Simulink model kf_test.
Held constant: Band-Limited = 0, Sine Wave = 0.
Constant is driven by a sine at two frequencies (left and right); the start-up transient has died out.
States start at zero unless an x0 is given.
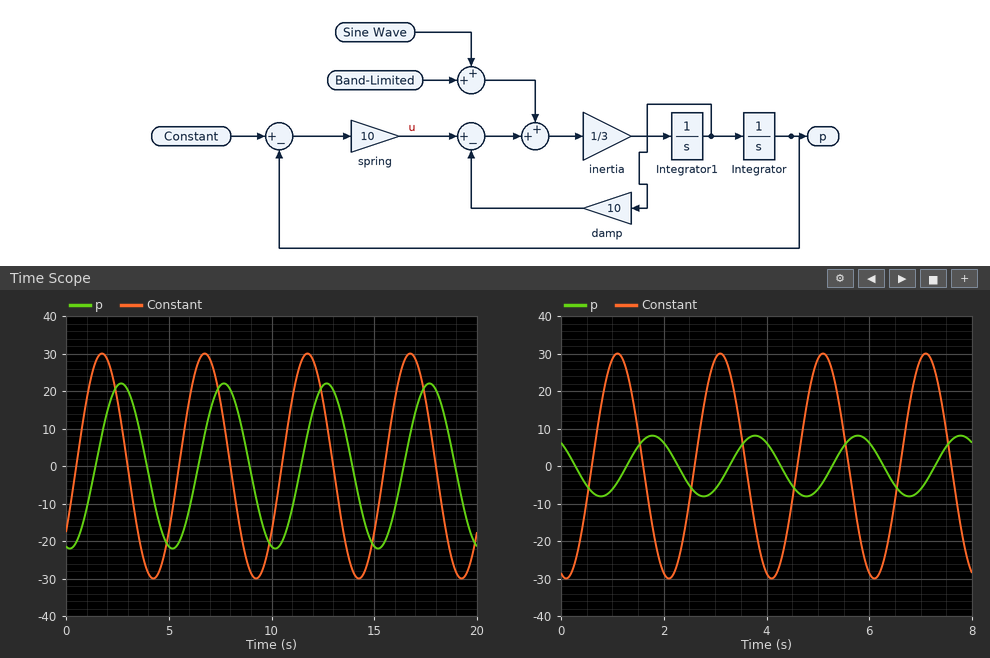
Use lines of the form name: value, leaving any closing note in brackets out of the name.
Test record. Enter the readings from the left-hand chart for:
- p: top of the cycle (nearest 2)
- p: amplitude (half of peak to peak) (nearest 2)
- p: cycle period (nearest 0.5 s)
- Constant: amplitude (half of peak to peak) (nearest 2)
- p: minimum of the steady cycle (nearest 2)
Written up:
p: top of the cycle: 22
p: amplitude (half of peak to peak): 22
p: cycle period: 5.0 s
Constant: amplitude (half of peak to peak): 30
p: minimum of the steady cycle: -22
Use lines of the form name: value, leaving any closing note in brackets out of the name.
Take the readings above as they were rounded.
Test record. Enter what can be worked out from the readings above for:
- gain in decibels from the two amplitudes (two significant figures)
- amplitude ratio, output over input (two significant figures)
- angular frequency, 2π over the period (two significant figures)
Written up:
gain in decibels from the two amplitudes: -2.7 dB
amplitude ratio, output over input: 0.73
angular frequency, 2π over the period: 1.3 rad/s
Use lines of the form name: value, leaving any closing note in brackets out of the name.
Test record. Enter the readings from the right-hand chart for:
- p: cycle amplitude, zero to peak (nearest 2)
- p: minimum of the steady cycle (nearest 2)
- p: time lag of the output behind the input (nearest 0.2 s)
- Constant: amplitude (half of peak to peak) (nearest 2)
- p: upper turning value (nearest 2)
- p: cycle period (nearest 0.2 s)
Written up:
p: cycle amplitude, zero to peak: 8
p: minimum of the steady cycle: -8
p: time lag of the output behind the input: 0.6 s
Constant: amplitude (half of peak to peak): 30
p: upper turning value: 8
p: cycle period: 2.0 s
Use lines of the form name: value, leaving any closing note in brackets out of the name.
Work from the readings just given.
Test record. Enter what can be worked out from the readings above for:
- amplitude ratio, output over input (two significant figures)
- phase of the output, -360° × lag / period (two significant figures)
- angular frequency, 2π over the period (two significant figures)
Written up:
amplitude ratio, output over input: 0.27
phase of the output, -360° × lag / period: -110°
angular frequency, 2π over the period: 3.1 rad/s
